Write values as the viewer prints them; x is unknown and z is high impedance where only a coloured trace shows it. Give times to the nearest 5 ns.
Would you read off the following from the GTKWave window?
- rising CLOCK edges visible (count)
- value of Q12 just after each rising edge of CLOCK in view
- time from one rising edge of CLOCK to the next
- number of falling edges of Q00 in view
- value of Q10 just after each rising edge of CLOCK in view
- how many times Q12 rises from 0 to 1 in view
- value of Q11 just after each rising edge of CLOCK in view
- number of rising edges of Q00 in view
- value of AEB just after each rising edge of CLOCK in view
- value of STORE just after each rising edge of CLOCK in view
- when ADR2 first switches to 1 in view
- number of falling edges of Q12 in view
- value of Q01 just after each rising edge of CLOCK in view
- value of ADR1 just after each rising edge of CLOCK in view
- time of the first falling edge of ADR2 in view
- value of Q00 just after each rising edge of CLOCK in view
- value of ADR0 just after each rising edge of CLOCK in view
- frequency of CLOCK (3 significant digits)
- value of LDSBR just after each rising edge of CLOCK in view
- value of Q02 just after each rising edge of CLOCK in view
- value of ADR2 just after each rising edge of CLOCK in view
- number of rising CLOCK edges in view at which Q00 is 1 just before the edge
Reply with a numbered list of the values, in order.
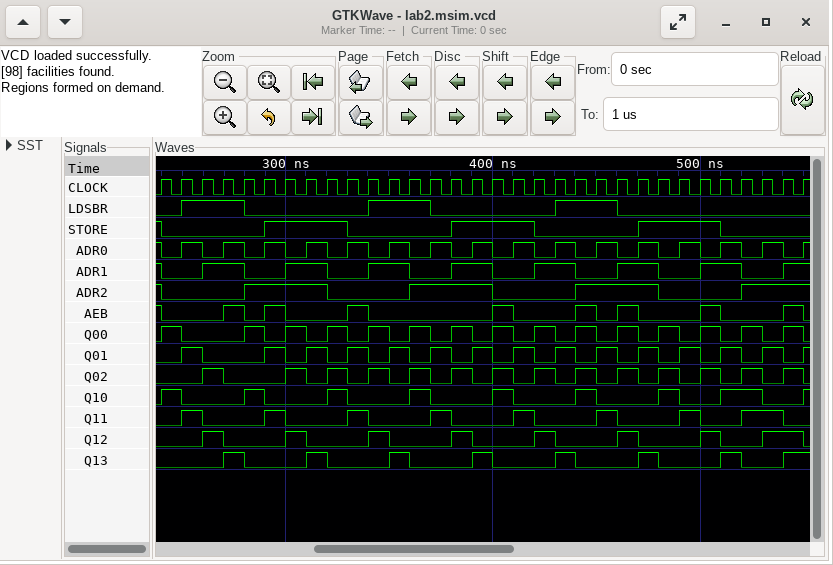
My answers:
1. 32
2. 0 0 1 0 0 0 1 0 0 0 1 0 0 0 1 0 0 0 1 0 0 0 1 0 0 0 1 0 0 1 1 0
3. 10 ns
4. 15
5. 1 0 0 0 1 0 0 0 1 0 0 0 1 0 0 0 1 0 0 0 1 0 0 0 1 0 0 1 1 0 0 1
6. 8
7. 0 1 0 0 0 1 0 0 0 1 0 0 0 1 0 0 0 1 0 0 0 1 0 0 0 1 0 0 1 1 0 0
8. 15
9. 0 0 0 1 0 1 0 0 0 1 0 0 0 0 0 0 1 0 0 0 1 0 1 0 0 0 1 0 0 0 1 0
10. 0 0 0 0 0 1 1 1 1 0 0 0 0 0 1 1 1 1 0 0 0 0 0 1 1 1 1 0 0 0 0 0
11. 280 ns
12. 8
13. 0 1 0 0 0 1 0 1 0 1 0 1 0 1 0 1 0 1 0 1 0 1 0 1 0 1 0 1 0 1 0 1
14. 0 0 1 1 0 0 1 1 0 0 1 1 0 0 1 1 0 0 1 1 0 0 1 1 0 0 1 1 0 0 1 1
15. 240 ns
16. 1 0 0 0 1 0 1 0 1 0 1 0 1 0 1 0 1 0 1 0 1 0 1 0 1 0 1 0 1 0 1 0
17. 0 1 0 1 0 1 0 1 0 1 0 1 0 1 0 1 0 1 0 1 0 1 0 1 0 1 0 1 0 1 0 1
18. 100 MHz
19. 0 1 1 1 0 0 0 0 0 0 1 1 1 0 0 0 0 0 0 1 1 1 0 0 0 0 0 0 0 0 0 0
20. 0 0 1 0 0 0 1 0 1 0 1 0 1 0 1 0 1 0 1 0 1 0 1 0 1 0 1 0 1 0 1 0
21. 0 0 0 0 1 1 1 1 0 0 0 0 1 1 1 1 0 0 0 0 1 1 1 1 0 0 0 0 1 1 1 1
22. 15
